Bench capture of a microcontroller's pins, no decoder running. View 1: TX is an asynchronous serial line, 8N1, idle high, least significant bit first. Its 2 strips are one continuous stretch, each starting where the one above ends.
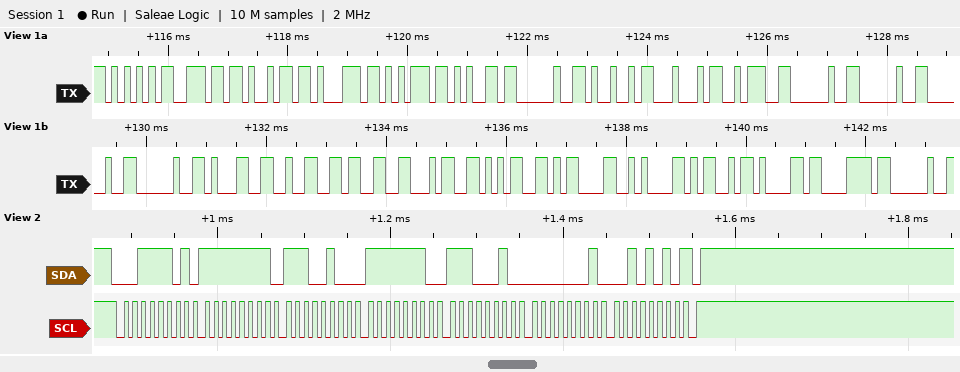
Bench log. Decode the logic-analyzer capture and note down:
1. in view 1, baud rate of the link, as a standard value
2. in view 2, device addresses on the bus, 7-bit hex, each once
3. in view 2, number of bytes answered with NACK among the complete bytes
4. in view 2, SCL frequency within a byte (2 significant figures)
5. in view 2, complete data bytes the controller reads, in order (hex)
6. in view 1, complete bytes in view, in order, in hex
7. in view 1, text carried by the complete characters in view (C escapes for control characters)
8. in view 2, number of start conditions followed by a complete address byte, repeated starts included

9600 baud
0x1E
1
100 kHz
FF E4 FE E2 01 2A
55 6E 69 71 75 65 20 49 44 3A 20 20 20 20 31 32 33 34 35 0D 0A 4D 61 78 20
"Unique ID:    12345\r\nMax "
1
